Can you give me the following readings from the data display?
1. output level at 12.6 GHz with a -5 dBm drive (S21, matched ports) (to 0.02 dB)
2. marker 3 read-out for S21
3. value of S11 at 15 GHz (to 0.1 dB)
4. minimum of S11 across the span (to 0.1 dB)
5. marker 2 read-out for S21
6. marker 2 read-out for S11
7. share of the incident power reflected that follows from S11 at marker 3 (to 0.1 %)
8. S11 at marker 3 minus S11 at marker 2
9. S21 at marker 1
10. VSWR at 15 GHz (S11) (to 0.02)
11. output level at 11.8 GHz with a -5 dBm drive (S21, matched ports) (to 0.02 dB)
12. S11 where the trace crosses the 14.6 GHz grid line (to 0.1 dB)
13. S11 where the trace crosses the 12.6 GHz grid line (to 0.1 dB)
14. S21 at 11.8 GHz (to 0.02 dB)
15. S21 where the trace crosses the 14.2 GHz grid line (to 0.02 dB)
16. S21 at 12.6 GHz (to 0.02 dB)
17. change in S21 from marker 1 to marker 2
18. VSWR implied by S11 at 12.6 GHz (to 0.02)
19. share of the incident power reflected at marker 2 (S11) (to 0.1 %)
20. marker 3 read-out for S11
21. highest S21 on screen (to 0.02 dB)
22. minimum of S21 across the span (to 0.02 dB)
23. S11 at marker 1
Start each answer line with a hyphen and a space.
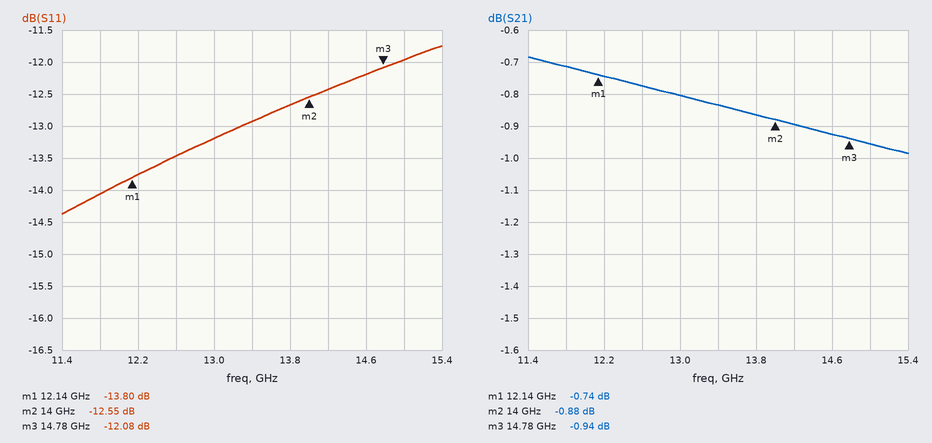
- -5.78 dBm
- -0.94 dB
- -12.0 dB
- -14.4 dB
- -0.88 dB
- -12.55 dB
- 6.2 %
- 0.47 dB
- -0.74 dB
- 1.68
- -5.72 dBm
- -12.2 dB
- -13.5 dB
- -0.72 dB
- -0.90 dB
- -0.78 dB
- -0.14 dB
- 1.54
- 5.6 %
- -12.08 dB
- -0.68 dB
- -0.98 dB
- -13.80 dB
